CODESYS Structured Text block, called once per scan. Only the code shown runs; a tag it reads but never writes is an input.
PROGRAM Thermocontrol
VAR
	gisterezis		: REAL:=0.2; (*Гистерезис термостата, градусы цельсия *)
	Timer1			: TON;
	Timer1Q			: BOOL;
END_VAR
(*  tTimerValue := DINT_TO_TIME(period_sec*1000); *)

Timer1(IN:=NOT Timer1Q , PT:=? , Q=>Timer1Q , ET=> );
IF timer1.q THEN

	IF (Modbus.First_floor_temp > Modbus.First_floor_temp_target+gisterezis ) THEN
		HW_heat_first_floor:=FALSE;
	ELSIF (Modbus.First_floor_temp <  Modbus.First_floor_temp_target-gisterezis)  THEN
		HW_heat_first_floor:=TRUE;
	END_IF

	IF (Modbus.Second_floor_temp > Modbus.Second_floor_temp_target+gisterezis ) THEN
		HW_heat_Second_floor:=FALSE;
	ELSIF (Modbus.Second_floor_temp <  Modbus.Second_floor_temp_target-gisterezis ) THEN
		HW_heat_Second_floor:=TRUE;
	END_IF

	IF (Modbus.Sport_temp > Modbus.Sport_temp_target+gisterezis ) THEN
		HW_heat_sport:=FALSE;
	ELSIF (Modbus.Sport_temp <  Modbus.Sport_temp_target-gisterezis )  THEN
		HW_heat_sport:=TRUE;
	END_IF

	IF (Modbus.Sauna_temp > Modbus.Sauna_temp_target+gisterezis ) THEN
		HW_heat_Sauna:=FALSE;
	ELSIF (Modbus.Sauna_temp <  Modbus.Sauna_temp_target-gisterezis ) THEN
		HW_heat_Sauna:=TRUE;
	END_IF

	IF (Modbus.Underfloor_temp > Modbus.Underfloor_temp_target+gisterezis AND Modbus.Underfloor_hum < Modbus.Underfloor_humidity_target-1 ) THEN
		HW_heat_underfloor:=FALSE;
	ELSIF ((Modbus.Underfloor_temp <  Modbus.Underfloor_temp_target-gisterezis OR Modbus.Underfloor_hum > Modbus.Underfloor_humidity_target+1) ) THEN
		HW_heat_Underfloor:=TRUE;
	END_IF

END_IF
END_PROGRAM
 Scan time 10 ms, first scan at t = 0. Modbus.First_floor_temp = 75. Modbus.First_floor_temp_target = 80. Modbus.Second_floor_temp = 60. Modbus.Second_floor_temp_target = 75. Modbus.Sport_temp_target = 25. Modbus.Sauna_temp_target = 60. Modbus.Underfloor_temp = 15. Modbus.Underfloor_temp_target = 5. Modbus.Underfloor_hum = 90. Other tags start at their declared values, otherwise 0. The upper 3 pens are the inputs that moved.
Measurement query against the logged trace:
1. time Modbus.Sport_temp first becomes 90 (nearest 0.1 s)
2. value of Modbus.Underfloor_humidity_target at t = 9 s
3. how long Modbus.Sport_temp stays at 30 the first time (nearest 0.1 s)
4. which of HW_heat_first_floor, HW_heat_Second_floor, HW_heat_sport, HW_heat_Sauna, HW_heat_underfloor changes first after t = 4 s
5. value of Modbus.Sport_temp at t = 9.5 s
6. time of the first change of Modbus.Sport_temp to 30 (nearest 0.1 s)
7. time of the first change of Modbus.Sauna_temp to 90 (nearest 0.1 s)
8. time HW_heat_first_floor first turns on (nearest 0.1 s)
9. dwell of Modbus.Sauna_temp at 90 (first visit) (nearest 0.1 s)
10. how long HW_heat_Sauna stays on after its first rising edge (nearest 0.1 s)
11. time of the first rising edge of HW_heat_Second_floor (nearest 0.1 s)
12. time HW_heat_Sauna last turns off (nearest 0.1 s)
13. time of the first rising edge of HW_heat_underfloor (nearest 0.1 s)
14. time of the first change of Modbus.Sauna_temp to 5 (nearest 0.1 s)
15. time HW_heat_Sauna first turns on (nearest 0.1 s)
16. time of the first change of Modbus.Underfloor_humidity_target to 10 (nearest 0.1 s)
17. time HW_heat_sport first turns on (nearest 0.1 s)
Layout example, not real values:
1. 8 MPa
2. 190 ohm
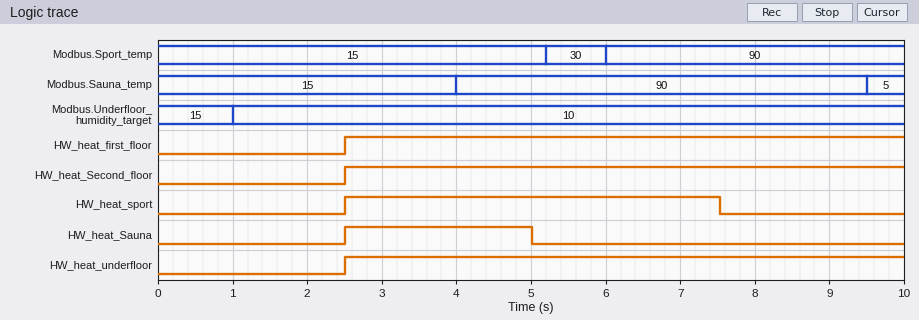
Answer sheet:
1. 6.0 s
2. 10
3. 0.8 s
4. HW_heat_Sauna
5. 90
6. 5.2 s
7. 4.0 s
8. 2.5 s
9. 5.5 s
10. 2.5 s
11. 2.5 s
12. 5.0 s
13. 2.5 s
14. 9.5 s
15. 2.5 s
16. 1.0 s
17. 2.5 s
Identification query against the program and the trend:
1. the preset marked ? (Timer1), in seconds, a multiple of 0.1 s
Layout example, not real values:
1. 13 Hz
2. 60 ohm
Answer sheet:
1. 2.5 s
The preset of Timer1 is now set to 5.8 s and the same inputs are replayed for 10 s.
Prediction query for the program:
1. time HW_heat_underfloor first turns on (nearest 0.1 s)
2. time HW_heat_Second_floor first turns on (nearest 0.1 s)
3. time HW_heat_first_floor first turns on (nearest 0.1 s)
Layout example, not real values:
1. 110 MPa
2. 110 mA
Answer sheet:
1. 5.8 s
2. 5.8 s
3. 5.8 s
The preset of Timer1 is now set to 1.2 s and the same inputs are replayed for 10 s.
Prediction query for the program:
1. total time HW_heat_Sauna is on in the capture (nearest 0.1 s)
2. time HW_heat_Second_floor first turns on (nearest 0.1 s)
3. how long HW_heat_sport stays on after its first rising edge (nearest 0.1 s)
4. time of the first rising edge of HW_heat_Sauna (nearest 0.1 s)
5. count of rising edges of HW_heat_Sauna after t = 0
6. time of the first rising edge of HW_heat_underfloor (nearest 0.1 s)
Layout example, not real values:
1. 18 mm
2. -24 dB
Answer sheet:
1. 3.9 s
2. 1.2 s
3. 4.9 s
4. 1.2 s
5. 2
6. 1.2 s
